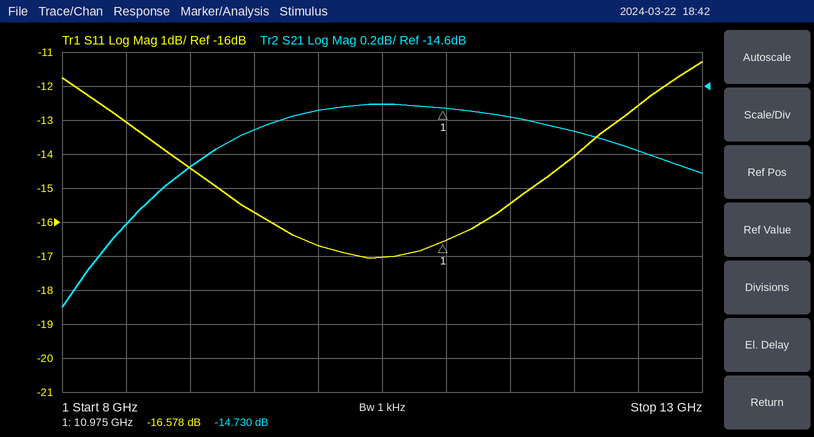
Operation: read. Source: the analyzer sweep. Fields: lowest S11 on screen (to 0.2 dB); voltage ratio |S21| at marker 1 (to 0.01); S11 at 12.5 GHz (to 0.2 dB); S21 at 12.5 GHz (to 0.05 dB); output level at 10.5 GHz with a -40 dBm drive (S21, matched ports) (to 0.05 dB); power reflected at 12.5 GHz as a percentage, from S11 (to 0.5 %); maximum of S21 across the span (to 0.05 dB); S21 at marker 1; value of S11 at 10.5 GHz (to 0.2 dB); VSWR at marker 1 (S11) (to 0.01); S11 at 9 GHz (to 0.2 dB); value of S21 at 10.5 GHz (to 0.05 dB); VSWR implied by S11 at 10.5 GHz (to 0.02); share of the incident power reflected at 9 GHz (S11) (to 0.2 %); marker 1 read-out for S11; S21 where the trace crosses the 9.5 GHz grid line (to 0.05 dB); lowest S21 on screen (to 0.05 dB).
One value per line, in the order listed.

-17.0 dB
0.18
-12.6 dB
-15.00 dB
-54.70 dBm
5.5 %
-14.70 dB
-14.730 dB
-17.0 dB
1.35
-14.4 dB
-14.70 dB
1.32
3.6 %
-16.578 dB
-14.85 dB
-15.90 dB
